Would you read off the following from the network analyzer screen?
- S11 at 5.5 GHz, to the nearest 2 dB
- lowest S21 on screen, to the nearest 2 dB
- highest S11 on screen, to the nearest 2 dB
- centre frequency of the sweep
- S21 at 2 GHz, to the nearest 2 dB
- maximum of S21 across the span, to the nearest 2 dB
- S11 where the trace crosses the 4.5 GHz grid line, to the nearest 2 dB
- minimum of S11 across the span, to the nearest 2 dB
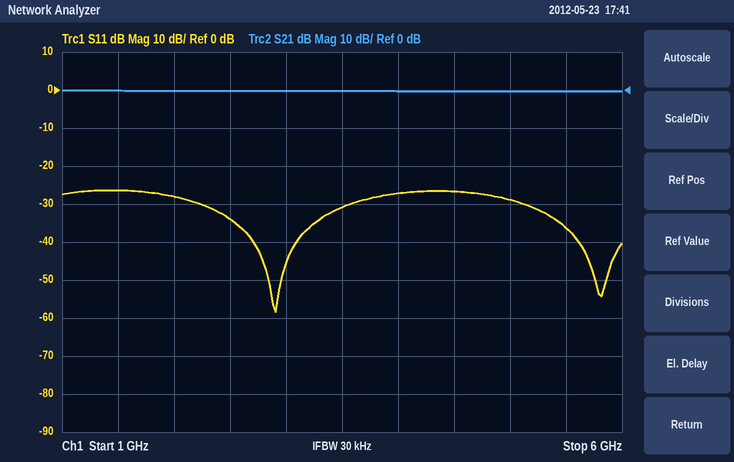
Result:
-36 dB
0 dB
-26 dB
3.5 GHz
0 dB
0 dB
-26 dB
-58 dB
